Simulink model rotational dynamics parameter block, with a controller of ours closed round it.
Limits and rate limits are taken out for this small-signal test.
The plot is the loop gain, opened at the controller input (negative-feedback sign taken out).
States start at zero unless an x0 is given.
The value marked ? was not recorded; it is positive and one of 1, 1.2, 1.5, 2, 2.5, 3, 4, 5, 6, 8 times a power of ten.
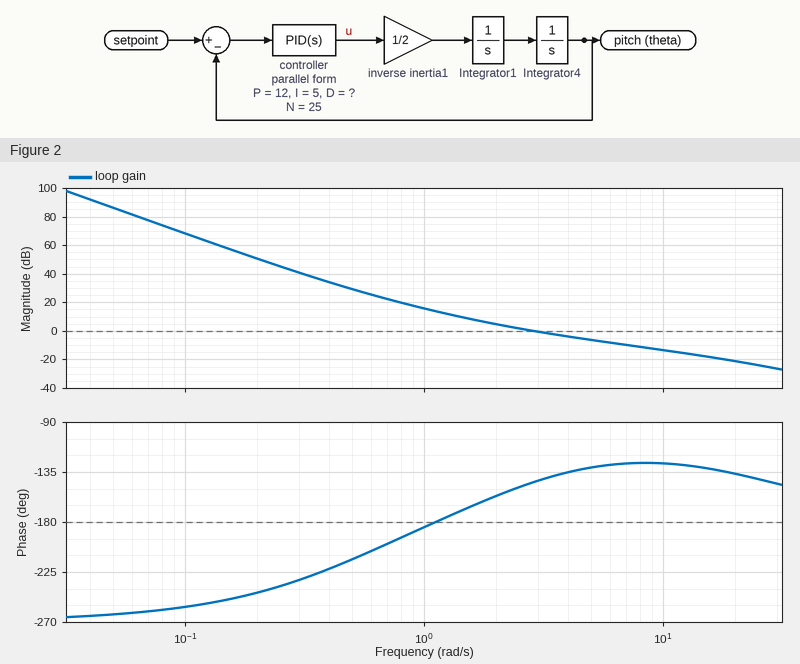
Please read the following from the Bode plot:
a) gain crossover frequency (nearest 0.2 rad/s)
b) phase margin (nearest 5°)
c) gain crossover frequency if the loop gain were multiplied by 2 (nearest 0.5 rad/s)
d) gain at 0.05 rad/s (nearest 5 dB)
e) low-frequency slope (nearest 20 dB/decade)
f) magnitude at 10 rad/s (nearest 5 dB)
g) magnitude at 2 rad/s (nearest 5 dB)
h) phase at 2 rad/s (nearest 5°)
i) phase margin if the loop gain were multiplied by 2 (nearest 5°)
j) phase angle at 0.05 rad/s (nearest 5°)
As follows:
2.8 rad/s
35°
5.0 rad/s
85 dB
-60 dB/decade
-15 dB
5 dB
-155°
50°
-265°
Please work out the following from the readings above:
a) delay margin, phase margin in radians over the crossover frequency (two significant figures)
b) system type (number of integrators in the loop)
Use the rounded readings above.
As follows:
0.22 s
3
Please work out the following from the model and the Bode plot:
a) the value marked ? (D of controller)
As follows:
4
